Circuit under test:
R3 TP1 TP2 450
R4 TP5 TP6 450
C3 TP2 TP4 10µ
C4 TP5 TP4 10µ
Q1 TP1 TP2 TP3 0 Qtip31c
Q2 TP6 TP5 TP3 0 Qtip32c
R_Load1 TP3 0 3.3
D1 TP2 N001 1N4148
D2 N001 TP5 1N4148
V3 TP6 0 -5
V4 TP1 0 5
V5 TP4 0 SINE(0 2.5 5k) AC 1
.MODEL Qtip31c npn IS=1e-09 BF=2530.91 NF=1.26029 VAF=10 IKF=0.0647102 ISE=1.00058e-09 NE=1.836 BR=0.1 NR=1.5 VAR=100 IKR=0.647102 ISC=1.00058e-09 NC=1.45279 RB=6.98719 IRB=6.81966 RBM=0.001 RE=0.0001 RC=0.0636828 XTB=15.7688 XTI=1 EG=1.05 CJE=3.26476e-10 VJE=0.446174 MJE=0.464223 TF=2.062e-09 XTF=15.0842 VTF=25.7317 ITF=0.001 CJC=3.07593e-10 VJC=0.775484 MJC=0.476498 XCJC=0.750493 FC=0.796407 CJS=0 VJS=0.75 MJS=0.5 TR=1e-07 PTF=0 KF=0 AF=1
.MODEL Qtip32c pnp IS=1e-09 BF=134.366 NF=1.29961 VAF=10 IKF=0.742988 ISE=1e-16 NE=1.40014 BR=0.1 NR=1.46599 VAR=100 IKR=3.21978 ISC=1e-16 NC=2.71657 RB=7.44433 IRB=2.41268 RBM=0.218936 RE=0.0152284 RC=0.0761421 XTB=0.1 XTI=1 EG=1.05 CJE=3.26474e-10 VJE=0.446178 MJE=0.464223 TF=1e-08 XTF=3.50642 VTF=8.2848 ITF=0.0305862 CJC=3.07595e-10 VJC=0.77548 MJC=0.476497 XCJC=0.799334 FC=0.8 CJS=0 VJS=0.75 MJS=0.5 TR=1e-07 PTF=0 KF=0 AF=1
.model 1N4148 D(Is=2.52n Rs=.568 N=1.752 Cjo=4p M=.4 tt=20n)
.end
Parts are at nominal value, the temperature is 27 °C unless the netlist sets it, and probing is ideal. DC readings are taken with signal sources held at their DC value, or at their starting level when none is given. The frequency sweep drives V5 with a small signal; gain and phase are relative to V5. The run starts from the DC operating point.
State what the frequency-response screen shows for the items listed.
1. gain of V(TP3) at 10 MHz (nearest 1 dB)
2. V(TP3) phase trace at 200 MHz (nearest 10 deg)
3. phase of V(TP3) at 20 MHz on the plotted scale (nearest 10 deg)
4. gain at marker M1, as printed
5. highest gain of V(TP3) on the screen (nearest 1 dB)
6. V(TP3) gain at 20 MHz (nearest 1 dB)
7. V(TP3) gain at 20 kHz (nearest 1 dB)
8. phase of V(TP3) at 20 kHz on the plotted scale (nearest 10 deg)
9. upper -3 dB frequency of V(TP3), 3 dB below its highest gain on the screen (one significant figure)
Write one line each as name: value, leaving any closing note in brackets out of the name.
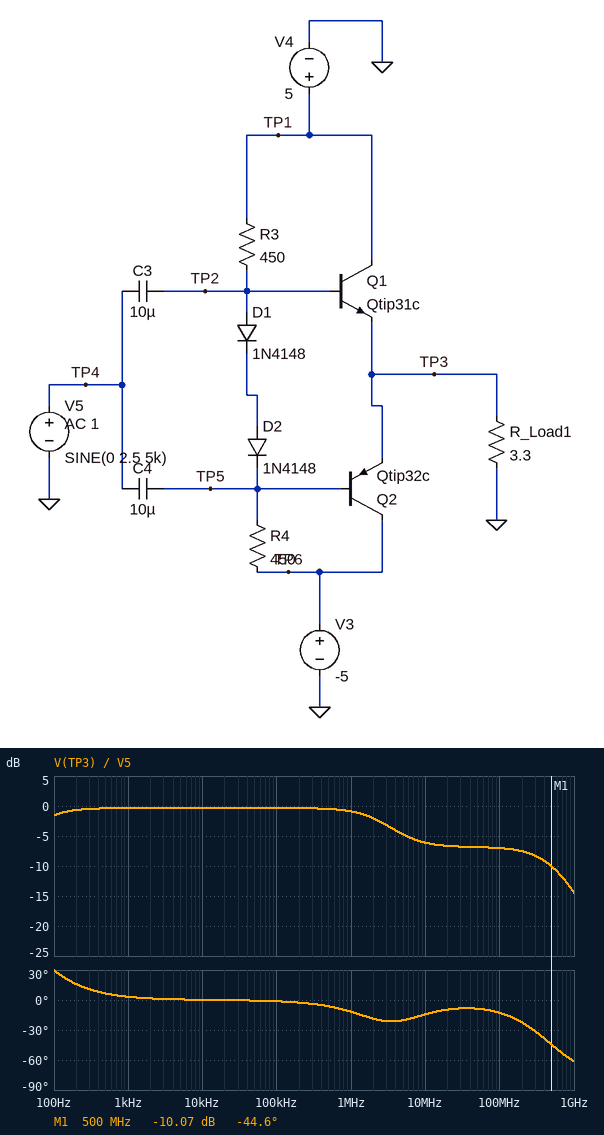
gain of V(TP3) at 10 MHz: -6 dB
V(TP3) phase trace at 200 MHz: -20 deg
phase of V(TP3) at 20 MHz on the plotted scale: -10 deg
gain at marker M1, as printed: -10.07 dB
highest gain of V(TP3) on the screen: 0 dB
V(TP3) gain at 20 MHz: -7 dB
V(TP3) gain at 20 kHz: 0 dB
phase of V(TP3) at 20 kHz on the plotted scale: 0 deg
upper -3 dB frequency of V(TP3), 3 dB below its highest gain on the screen: 3 MHz
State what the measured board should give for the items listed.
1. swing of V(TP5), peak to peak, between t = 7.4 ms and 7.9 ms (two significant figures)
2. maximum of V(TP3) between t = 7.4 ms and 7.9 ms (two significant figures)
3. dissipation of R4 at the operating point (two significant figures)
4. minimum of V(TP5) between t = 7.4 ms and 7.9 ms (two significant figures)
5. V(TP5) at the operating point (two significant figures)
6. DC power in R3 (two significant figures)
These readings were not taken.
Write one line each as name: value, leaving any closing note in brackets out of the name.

swing of V(TP5), peak to peak, between t = 7.4 ms and 7.9 ms: 5.0 V
maximum of V(TP3) between t = 7.4 ms and 7.9 ms: 2.4 V
dissipation of R4 at the operating point: 42 mW
minimum of V(TP5) between t = 7.4 ms and 7.9 ms: -3.1 V
V(TP5) at the operating point: -640 mV
DC power in R3: 41 mW
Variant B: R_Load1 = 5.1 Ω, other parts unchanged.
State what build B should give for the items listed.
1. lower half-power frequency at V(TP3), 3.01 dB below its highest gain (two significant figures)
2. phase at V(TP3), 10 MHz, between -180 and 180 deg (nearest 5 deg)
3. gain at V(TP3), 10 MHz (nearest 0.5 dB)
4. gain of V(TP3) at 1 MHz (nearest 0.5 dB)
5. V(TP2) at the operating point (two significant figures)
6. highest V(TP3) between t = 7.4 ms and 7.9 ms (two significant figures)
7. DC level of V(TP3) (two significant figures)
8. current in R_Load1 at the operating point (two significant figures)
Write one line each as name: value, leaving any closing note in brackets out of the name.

lower half-power frequency at V(TP3), 3.01 dB below its highest gain: 50 Hz
phase at V(TP3), 10 MHz, between -180 and 180 deg: -10 deg
gain at V(TP3), 10 MHz: -4.5 dB
gain of V(TP3) at 1 MHz: -0.5 dB
V(TP2) at the operating point: 720 mV
highest V(TP3) between t = 7.4 ms and 7.9 ms: 2.5 V
DC level of V(TP3): 36 mV
current in R_Load1 at the operating point: 7.0 mA
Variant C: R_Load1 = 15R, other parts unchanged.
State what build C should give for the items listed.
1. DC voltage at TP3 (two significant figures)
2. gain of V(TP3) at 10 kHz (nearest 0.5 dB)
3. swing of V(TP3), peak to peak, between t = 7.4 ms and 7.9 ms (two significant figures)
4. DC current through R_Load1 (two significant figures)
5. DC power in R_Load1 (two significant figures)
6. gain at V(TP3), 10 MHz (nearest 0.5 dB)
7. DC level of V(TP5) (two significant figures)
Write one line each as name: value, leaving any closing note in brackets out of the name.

DC voltage at TP3: 43 mV
gain of V(TP3) at 10 kHz: 0 dB
swing of V(TP3), peak to peak, between t = 7.4 ms and 7.9 ms: 4.9 V
DC current through R_Load1: 2.9 mA
DC power in R_Load1: 120 µW
gain at V(TP3), 10 MHz: -2.0 dB
DC level of V(TP5): -630 mV
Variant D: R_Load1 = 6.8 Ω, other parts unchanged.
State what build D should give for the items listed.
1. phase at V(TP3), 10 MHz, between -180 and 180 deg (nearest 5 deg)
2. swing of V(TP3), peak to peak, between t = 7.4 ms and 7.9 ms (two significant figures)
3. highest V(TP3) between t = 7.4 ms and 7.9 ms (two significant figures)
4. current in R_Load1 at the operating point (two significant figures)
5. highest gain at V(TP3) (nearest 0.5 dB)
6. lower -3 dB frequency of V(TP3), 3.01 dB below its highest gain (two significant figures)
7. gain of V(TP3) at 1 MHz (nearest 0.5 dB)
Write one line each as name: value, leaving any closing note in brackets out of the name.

phase at V(TP3), 10 MHz, between -180 and 180 deg: -10 deg
swing of V(TP3), peak to peak, between t = 7.4 ms and 7.9 ms: 4.9 V
highest V(TP3) between t = 7.4 ms and 7.9 ms: 2.5 V
current in R_Load1 at the operating point: 5.6 mA
highest gain at V(TP3): 0 dB
lower -3 dB frequency of V(TP3), 3.01 dB below its highest gain: 47 Hz
gain of V(TP3) at 1 MHz: -0.5 dB
